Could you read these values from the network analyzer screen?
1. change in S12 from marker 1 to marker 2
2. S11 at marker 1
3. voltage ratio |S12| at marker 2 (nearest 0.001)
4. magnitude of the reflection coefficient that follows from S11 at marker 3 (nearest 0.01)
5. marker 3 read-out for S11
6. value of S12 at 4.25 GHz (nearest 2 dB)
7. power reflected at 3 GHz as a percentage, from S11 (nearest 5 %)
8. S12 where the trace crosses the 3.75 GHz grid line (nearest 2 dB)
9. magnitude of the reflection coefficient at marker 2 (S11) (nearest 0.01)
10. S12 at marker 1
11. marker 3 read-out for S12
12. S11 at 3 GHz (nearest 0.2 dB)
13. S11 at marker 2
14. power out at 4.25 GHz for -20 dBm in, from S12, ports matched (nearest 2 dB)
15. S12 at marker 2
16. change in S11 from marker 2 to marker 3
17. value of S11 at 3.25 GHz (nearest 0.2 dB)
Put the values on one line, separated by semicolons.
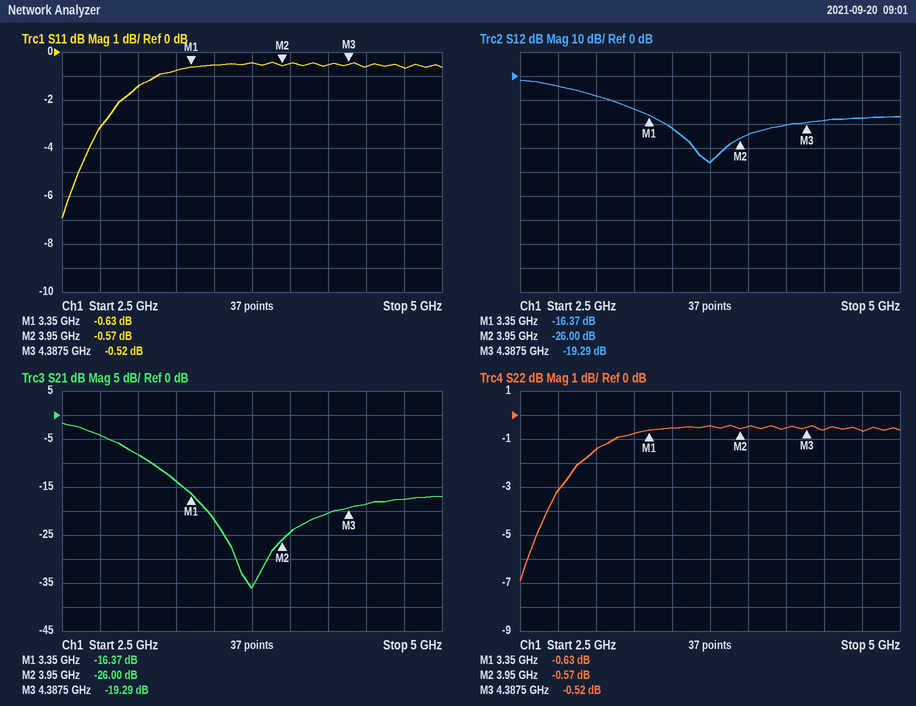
-9.63 dB; -0.63 dB; 0.050; 0.94; -0.52 dB; -20 dB; 70 %; -36 dB; 0.94; -16.37 dB; -19.29 dB; -1.4 dB; -0.57 dB; -40 dBm; -26.00 dB; 0.05 dB; -0.8 dB
